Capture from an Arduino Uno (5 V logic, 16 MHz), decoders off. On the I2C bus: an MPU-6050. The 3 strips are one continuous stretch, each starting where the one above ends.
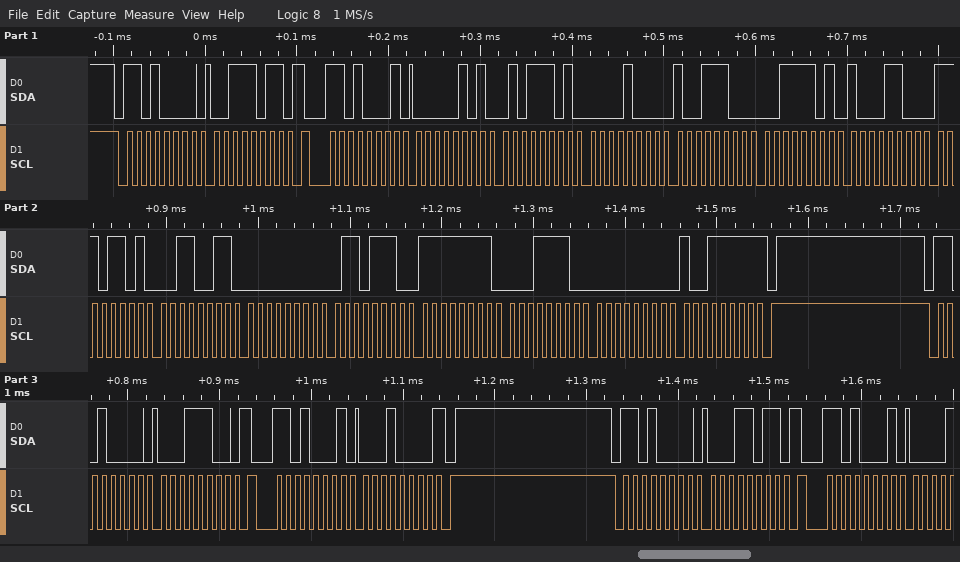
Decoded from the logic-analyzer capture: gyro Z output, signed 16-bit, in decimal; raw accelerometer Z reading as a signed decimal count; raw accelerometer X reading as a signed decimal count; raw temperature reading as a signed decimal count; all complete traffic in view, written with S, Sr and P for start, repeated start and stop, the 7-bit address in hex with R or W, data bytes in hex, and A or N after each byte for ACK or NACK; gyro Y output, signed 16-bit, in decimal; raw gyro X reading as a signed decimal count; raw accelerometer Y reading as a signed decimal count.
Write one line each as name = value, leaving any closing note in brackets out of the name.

gyro Z output, signed 16-bit, in decimal = 159
raw accelerometer Z reading as a signed decimal count = 15756
raw accelerometer X reading as a signed decimal count = 1373
raw temperature reading as a signed decimal count = -4813
all complete traffic in view, written with S, Sr and P for start, repeated start and stop, the 7-bit address in hex with R or W, data bytes in hex, and A or N after each byte for ACK or NACK = S 68W A 3B A Sr 68R A 05 A 5D A 08 A 9C A 3D A 8C A ED A 33 A 00 A 6E A FF A 1E A 00 A 9F N P S 68W A 1C A Sr 68R A 10 N P S 68W A 1B A Sr 68R A
gyro Y output, signed 16-bit, in decimal = -226
raw gyro X reading as a signed decimal count = 110
raw accelerometer Y reading as a signed decimal count = 2204
